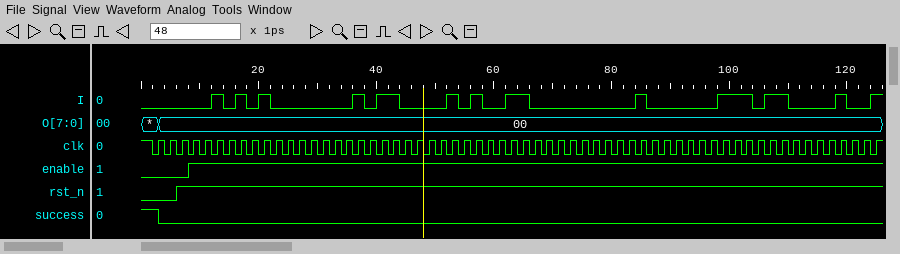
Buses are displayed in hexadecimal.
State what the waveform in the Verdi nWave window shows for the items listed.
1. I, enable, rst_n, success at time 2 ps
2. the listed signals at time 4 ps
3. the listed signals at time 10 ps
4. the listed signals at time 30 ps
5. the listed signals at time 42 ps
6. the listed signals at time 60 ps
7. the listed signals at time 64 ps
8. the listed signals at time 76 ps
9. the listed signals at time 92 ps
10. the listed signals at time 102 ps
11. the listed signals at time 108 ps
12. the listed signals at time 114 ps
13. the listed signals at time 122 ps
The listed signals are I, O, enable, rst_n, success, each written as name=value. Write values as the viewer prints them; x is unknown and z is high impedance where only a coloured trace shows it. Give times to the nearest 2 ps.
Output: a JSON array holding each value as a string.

["I=0, enable=0, rst_n=0, success=1", "I=0, O=00, enable=0, rst_n=0, success=0", "I=0, O=00, enable=1, rst_n=1, success=0", "I=0, O=00, enable=1, rst_n=1, success=0", "I=1, O=00, enable=1, rst_n=1, success=0", "I=0, O=00, enable=1, rst_n=1, success=0", "I=1, O=00, enable=1, rst_n=1, success=0", "I=0, O=00, enable=1, rst_n=1, success=0", "I=0, O=00, enable=1, rst_n=1, success=0", "I=1, O=00, enable=1, rst_n=1, success=0", "I=1, O=00, enable=1, rst_n=1, success=0", "I=0, O=00, enable=1, rst_n=1, success=0", "I=0, O=00, enable=1, rst_n=1, success=0"]
